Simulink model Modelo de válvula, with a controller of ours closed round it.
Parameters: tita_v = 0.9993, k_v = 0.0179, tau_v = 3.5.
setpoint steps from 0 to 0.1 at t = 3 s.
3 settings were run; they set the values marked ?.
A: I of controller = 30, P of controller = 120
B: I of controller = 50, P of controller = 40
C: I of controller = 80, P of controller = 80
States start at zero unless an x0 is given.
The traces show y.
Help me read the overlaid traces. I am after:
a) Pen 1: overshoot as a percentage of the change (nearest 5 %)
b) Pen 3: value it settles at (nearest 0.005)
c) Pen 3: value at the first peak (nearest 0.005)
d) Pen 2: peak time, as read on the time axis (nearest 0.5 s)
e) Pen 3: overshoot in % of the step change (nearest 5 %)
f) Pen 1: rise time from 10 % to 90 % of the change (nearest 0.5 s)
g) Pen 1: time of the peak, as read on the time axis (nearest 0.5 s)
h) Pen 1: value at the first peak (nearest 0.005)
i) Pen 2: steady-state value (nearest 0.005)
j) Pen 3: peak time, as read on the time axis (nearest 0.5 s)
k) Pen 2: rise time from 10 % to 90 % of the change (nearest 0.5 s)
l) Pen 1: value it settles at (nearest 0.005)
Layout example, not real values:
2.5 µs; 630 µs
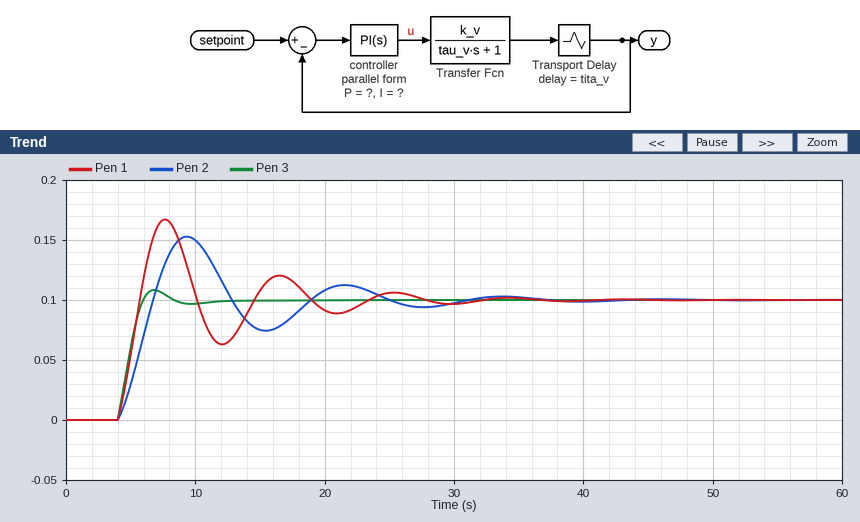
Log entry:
65 %; 0.100; 0.110; 9.5 s; 10 %; 1.5 s; 7.5 s; 0.165; 0.100; 7.0 s; 2.0 s; 0.100
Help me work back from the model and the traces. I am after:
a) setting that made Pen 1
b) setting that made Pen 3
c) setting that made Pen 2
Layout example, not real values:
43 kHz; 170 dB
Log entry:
C; A; B
